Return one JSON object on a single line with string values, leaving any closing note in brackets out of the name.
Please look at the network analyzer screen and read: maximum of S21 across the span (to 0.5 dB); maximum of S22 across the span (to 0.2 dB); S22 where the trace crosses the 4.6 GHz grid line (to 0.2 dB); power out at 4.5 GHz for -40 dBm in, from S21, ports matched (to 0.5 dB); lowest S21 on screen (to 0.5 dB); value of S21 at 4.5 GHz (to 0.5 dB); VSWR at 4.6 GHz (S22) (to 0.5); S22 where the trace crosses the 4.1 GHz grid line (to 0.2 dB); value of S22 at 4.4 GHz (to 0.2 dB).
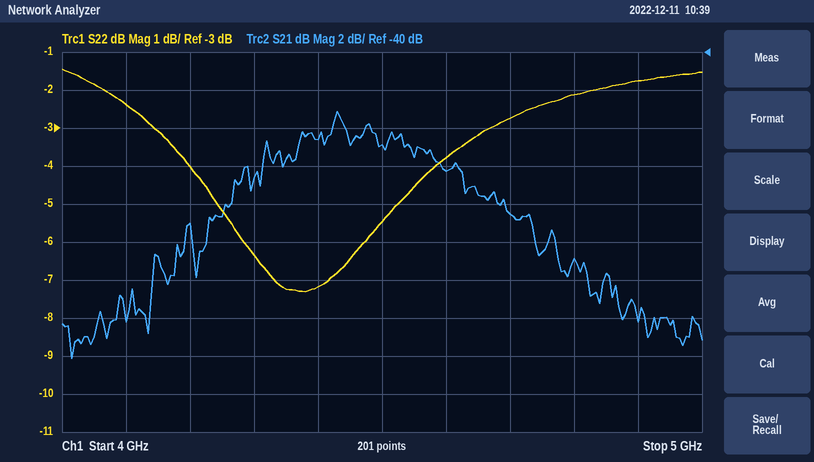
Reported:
{"maximum of S21 across the span": "-43.0 dB", "maximum of S22 across the span": "-1.4 dB", "S22 where the trace crosses the 4.6 GHz grid line": "-3.8 dB", "power out at 4.5 GHz for -40 dBm in, from S21, ports matched": "-85.0 dBm", "lowest S21 on screen": "-56.0 dB", "value of S21 at 4.5 GHz": "-45.0 dB", "VSWR at 4.6 GHz (S22)": "4.5", "S22 where the trace crosses the 4.1 GHz grid line": "-2.4 dB", "value of S22 at 4.4 GHz": "-7.2 dB"}
